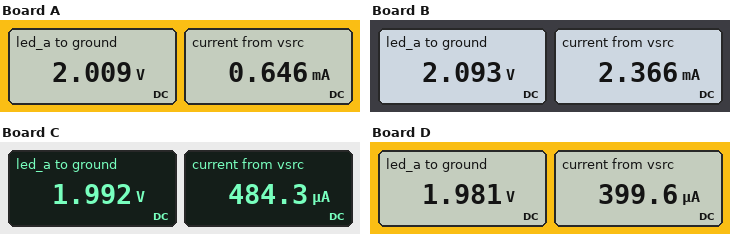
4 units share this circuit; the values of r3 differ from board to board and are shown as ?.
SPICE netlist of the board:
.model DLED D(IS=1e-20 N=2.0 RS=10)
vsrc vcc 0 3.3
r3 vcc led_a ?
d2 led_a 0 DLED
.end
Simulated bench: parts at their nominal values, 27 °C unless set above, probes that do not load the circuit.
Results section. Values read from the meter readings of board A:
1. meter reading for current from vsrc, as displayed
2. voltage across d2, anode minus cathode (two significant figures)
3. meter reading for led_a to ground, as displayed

0.646 mA
2.0 V
2.009 V
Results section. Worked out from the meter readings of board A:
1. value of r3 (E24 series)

2 kΩ
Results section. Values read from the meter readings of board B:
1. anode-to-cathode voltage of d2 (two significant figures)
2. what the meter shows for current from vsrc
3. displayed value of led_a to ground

2.1 V
2.366 mA
2.093 V
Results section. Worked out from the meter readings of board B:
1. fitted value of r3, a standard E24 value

510 Ω
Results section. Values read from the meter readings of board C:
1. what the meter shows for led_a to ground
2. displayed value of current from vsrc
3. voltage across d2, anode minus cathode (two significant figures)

1.992 V
484.3 µA
2.0 V
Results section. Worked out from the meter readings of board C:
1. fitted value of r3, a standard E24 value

2.7 kΩ
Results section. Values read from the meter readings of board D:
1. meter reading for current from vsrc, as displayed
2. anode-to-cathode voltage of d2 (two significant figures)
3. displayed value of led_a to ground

399.6 µA
2.0 V
1.981 V
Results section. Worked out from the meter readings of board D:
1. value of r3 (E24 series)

3.3 kΩ
